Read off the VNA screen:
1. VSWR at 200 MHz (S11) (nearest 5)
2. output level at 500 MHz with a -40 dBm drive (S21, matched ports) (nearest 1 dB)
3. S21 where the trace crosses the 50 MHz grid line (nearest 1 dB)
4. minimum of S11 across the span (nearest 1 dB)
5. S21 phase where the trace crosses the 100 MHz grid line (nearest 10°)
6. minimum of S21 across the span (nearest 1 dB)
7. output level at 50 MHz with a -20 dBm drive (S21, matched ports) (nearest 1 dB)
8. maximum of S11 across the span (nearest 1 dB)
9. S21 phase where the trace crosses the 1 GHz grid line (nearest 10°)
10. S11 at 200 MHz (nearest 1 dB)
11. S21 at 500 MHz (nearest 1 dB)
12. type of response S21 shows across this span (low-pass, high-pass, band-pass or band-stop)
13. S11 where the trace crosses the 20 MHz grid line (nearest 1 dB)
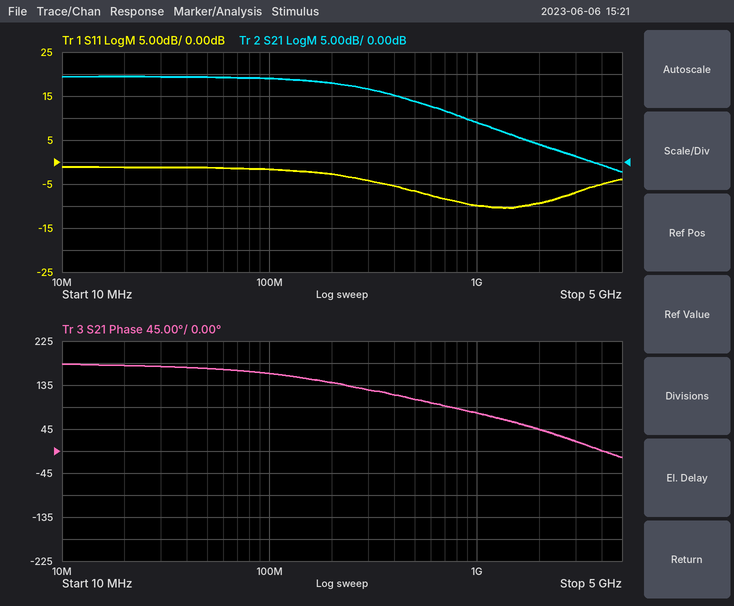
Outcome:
5
-26 dBm
19 dB
-10 dB
160°
-2 dB
-1 dBm
-1 dB
80°
-3 dB
14 dB
low-pass
-1 dB
